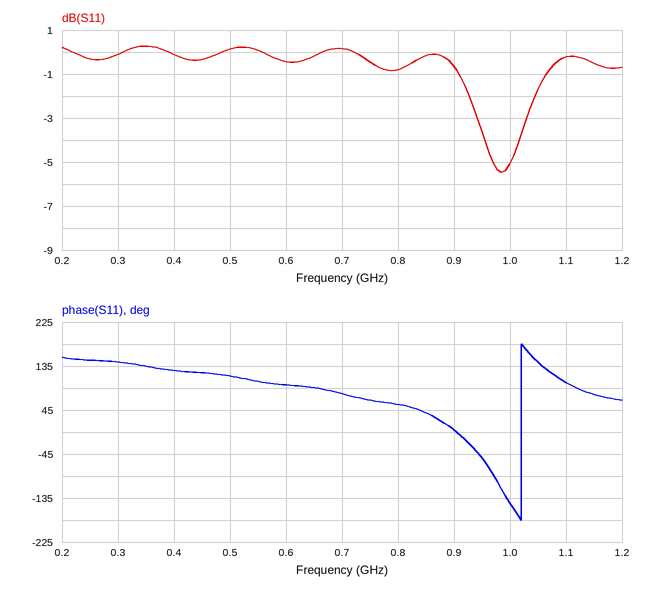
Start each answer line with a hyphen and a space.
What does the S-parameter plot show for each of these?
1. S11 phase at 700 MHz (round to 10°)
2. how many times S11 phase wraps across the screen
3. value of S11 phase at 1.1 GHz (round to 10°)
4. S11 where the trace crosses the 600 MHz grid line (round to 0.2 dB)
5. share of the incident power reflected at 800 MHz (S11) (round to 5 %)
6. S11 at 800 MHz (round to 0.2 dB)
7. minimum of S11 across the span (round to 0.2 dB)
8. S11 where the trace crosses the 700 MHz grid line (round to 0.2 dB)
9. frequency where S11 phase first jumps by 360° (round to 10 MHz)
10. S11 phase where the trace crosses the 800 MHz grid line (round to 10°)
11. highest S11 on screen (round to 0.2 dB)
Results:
- 80°
- 1
- 100°
- -0.4 dB
- 85 %
- -0.8 dB
- -5.4 dB
- 0.2 dB
- 1.02 GHz
- 60°
- 0.2 dB
